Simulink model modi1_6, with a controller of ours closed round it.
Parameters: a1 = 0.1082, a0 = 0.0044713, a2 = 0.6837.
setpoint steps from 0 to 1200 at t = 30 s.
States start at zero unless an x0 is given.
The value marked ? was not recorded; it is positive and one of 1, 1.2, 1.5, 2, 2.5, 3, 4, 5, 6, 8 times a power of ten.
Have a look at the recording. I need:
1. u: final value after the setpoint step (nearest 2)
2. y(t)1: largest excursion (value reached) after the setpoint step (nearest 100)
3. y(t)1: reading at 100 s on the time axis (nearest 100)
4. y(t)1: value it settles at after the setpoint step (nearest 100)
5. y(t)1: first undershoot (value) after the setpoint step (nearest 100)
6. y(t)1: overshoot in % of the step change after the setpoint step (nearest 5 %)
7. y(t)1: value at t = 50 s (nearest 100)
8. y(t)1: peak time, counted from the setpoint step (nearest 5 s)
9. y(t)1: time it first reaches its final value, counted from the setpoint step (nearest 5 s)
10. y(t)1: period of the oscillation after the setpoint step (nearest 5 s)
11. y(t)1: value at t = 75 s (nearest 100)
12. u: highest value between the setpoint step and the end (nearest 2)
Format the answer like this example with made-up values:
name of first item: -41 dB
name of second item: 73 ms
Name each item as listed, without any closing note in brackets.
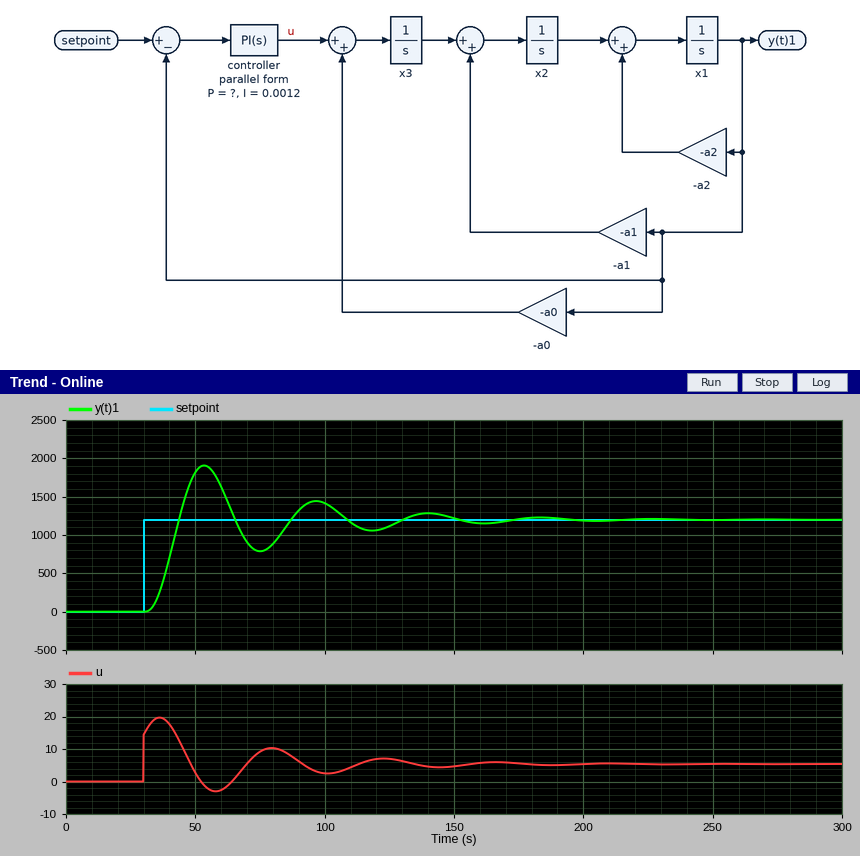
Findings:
u: final value after the setpoint step: 6
y(t)1: largest excursion (value reached) after the setpoint step: 1900
y(t)1: reading at 100 s on the time axis: 1400
y(t)1: value it settles at after the setpoint step: 1200
y(t)1: first undershoot (value) after the setpoint step: 800
y(t)1: overshoot in % of the step change after the setpoint step: 60 %
y(t)1: value at t = 50 s: 1800
y(t)1: peak time, counted from the setpoint step: 25 s
y(t)1: time it first reaches its final value, counted from the setpoint step: 15 s
y(t)1: period of the oscillation after the setpoint step: 45 s
y(t)1: value at t = 75 s: 800
u: highest value between the setpoint step and the end: 20
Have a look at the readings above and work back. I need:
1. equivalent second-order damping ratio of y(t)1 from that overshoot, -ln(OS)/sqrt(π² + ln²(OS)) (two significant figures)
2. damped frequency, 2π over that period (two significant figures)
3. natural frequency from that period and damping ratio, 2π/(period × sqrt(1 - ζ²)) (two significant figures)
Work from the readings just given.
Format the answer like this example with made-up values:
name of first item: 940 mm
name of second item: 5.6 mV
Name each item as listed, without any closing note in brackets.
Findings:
equivalent second-order damping ratio of y(t)1 from that overshoot, -ln(OS)/sqrt(π² + ln²(OS)): 0.16
damped frequency, 2π over that period: 0.14 rad/s
natural frequency from that period and damping ratio, 2π/(period × sqrt(1 - ζ²)): 0.14 rad/s
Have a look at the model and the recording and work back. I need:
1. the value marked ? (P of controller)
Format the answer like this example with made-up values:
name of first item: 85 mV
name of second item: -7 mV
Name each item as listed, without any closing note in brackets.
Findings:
the value marked ?: 0.012
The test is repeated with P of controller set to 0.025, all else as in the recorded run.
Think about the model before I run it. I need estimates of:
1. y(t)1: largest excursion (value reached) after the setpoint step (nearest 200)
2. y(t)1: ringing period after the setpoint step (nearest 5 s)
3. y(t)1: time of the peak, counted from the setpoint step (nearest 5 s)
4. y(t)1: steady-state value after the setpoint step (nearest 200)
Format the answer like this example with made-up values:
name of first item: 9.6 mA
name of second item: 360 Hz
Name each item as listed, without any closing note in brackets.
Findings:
y(t)1: largest excursion (value reached) after the setpoint step: 1800
y(t)1: ringing period after the setpoint step: 30 s
y(t)1: time of the peak, counted from the setpoint step: 15 s
y(t)1: steady-state value after the setpoint step: 1200
